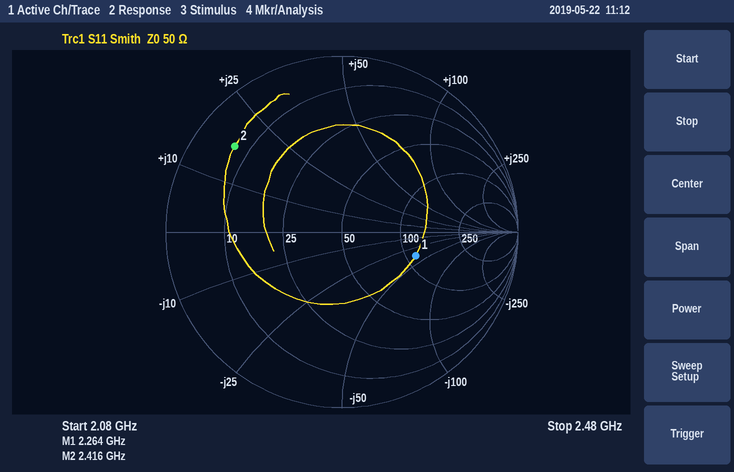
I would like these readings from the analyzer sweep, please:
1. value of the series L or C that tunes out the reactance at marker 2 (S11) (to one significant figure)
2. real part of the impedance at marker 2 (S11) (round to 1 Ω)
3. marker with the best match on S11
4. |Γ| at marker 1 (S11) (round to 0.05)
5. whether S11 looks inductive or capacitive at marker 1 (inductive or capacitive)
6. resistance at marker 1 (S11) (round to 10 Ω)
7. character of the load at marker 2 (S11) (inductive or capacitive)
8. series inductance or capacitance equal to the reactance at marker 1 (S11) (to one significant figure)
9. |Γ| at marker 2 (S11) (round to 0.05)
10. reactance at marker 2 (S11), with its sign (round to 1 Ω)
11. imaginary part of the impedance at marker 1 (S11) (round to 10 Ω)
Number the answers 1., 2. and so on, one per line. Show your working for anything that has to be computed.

1. C = 1/(2π × 2.416 GHz × 17 Ω) ≈ 4 pF
2. 7 Ω
3. marker 1
4. 0.45
5. capacitive
6. 110 Ω
7. inductive
8. C = 1/(2π × 2.264 GHz × 40 Ω) ≈ 2 pF
9. 0.80
10. +17 Ω
11. -40 Ω
